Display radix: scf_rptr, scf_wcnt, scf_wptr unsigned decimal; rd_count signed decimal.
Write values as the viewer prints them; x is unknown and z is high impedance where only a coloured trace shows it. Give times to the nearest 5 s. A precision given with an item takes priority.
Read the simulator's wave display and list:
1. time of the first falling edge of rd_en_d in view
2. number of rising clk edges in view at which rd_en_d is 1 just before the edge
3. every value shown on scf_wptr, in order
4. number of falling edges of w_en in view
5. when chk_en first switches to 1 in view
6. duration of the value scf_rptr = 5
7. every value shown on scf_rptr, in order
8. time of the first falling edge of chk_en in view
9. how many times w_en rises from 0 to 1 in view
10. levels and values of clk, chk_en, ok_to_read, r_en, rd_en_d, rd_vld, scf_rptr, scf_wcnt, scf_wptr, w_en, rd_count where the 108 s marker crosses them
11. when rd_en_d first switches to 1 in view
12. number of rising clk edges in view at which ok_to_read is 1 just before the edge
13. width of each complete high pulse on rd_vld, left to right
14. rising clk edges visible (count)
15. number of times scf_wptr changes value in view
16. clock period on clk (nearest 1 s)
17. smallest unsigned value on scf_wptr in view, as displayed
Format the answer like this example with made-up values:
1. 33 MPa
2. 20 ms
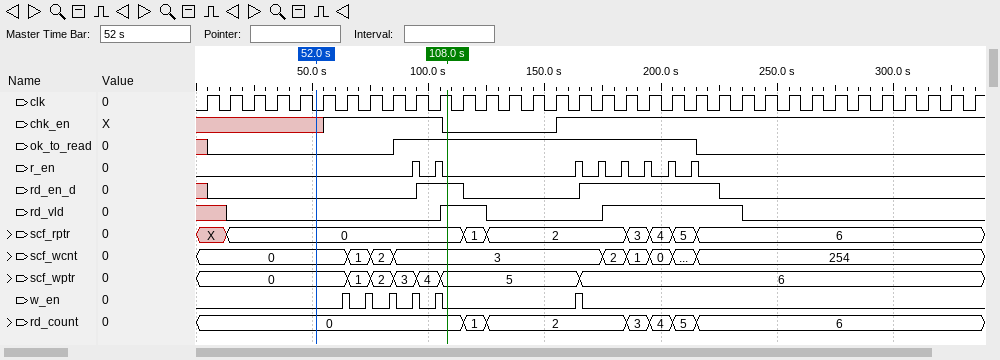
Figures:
1. 115 s
2. 8
3. 0, 1, 2, 3, 4, 5, 6
4. 6
5. 55 s
6. 10 s
7. X, 0, 1, 2, 3, 4, 5, 6
8. 105 s
9. 6
10. clk=1, chk_en=0, ok_to_read=1, r_en=0, rd_en_d=1, rd_vld=1, scf_rptr=0, scf_wcnt=3, scf_wptr=5, w_en=0, rd_count=0
11. 95 s
12. 13
13. 20 s, 60 s
14. 34
15. 6
16. 10 s
17. 0
